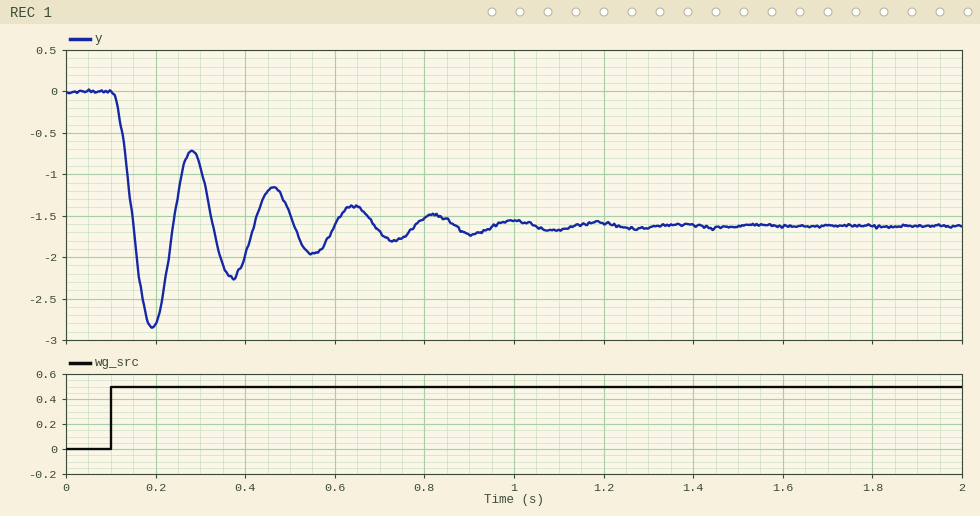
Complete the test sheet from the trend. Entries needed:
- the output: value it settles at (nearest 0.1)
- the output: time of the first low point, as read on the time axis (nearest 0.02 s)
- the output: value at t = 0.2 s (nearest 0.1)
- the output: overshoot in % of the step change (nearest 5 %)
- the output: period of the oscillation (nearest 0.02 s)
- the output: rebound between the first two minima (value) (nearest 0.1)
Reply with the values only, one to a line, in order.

-1.6
0.20 s
-2.8
75 %
0.18 s
-0.7
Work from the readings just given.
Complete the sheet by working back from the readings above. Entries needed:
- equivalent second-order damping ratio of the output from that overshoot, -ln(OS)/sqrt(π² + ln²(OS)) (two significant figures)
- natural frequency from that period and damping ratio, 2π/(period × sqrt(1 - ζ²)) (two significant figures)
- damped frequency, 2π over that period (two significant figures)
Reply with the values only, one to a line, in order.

0.091
35 rad/s
35 rad/s
